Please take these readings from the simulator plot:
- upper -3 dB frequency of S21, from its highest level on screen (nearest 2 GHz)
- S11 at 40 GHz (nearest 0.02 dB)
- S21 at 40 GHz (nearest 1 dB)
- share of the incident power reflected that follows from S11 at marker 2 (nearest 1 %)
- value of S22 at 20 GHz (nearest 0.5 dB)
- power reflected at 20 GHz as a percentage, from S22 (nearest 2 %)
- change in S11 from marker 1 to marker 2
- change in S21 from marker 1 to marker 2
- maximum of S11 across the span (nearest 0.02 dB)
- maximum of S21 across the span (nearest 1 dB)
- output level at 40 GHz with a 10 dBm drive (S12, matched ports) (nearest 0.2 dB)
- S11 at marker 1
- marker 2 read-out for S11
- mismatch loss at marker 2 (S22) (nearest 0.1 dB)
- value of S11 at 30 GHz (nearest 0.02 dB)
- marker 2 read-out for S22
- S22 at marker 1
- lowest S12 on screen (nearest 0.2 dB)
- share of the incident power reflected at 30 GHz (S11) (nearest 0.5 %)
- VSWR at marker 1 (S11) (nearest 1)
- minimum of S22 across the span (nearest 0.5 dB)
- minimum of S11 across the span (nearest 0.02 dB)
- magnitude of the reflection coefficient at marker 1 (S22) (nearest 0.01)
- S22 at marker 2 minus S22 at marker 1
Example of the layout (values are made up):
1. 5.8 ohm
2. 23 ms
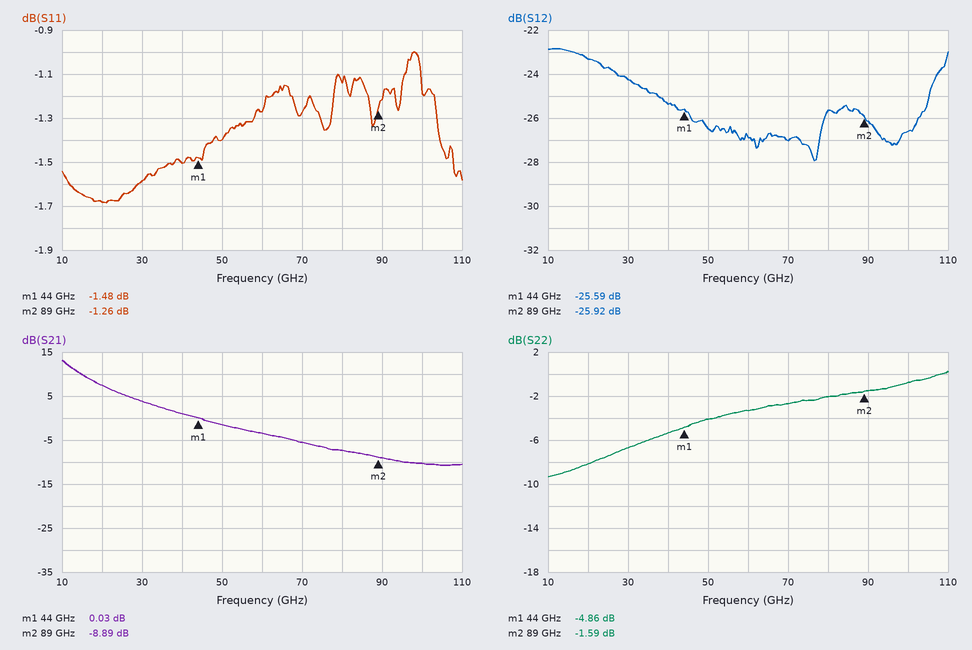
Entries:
1. 14 GHz
2. -1.50 dB
3. 1 dB
4. 75 %
5. -8.0 dB
6. 16 %
7. 0.22 dB
8. -8.92 dB
9. -1.00 dB
10. 13 dB
11. -15.4 dBm
12. -1.48 dB
13. -1.26 dB
14. 5.1 dB
15. -1.58 dB
16. -1.59 dB
17. -4.86 dB
18. -28.0 dB
19. 69.5 %
20. 12
21. -9.5 dB
22. -1.68 dB
23. 0.57
24. 3.27 dB
